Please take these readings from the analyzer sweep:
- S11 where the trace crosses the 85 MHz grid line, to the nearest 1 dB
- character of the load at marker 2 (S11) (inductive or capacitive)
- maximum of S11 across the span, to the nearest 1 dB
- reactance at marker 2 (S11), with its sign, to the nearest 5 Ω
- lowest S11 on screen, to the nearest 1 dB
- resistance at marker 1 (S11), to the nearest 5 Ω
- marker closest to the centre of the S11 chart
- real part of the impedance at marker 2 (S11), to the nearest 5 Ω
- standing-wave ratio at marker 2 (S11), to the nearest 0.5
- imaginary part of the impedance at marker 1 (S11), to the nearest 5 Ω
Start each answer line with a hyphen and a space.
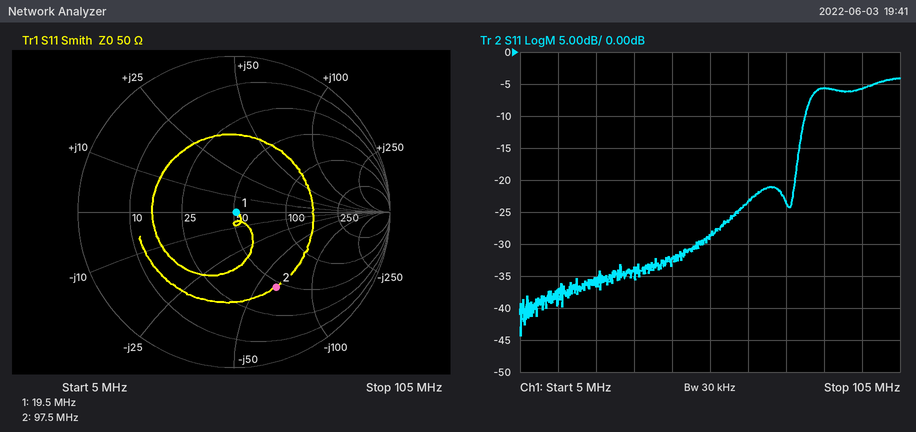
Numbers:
- -6 dB
- capacitive
- -4 dB
- -65 Ω
- -44 dB
- 50 Ω
- marker 1
- 45 Ω
- 3.5
- 0 Ω
